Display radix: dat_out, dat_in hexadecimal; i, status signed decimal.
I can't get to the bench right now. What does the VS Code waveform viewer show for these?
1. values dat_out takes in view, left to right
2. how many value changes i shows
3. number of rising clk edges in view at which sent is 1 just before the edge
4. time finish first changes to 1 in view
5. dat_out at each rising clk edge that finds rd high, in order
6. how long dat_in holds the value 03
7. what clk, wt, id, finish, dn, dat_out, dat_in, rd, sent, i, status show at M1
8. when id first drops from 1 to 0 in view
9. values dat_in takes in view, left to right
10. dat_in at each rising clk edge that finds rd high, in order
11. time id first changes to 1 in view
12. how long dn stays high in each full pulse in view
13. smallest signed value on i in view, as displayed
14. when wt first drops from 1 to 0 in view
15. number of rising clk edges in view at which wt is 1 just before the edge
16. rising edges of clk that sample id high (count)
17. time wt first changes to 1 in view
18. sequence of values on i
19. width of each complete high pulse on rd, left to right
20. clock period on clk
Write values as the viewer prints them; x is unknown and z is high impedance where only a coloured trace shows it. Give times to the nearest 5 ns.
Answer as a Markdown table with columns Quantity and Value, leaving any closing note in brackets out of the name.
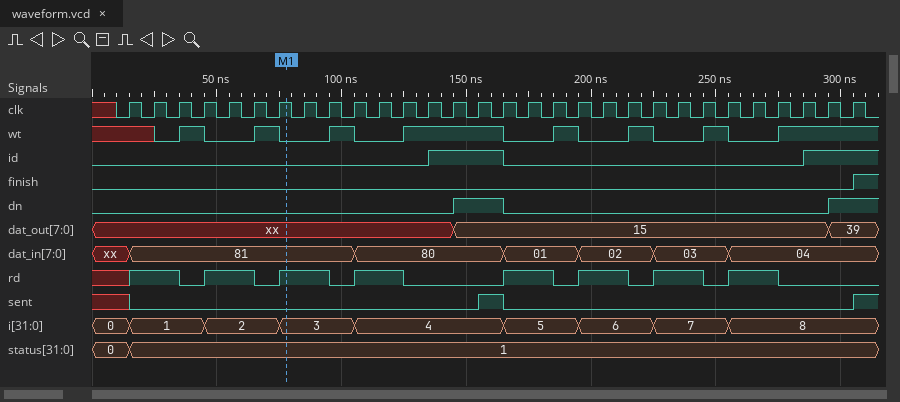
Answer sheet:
| Quantity | Value |
|---|---|
| values dat_out takes in view, left to right | xx, 15, 39 |
| how many value changes i shows | 8 |
| number of rising clk edges in view at which sent is 1 just before the edge | 1 |
| time finish first changes to 1 in view | 305 ns |
| dat_out at each rising clk edge that finds rd high, in order | xx, xx, xx, xx, xx, xx, xx, xx, 15, 15, 15, 15, 15, 15, 15, 15 |
| how long dat_in holds the value 03 | 30 ns |
| what clk, wt, id, finish, dn, dat_out, dat_in, rd, sent, i, status show at M1 | clk=1, wt=0, id=0, finish=0, dn=0, dat_out=xx, dat_in=81, rd=1, sent=0, i=3, status=1 |
| when id first drops from 1 to 0 in view | 165 ns |
| values dat_in takes in view, left to right | xx, 81, 80, 01, 02, 03, 04 |
| dat_in at each rising clk edge that finds rd high, in order | 81, 81, 81, 81, 81, 81, 80, 80, 01, 01, 02, 02, 03, 03, 04, 04 |
| time id first changes to 1 in view | 135 ns |
| how long dn stays high in each full pulse in view | 20 ns |
| smallest signed value on i in view, as displayed | 0 |
| when wt first drops from 1 to 0 in view | 45 ns |
| number of rising clk edges in view at which wt is 1 just before the edge | 13 |
| rising edges of clk that sample id high | 5 |
| time wt first changes to 1 in view | 35 ns |
| sequence of values on i | 0, 1, 2, 3, 4, 5, 6, 7, 8 |
| width of each complete high pulse on rd, left to right | 20 ns, 20 ns, 20 ns, 20 ns, 20 ns, 20 ns, 20 ns |
| clock period on clk | 10 ns |
